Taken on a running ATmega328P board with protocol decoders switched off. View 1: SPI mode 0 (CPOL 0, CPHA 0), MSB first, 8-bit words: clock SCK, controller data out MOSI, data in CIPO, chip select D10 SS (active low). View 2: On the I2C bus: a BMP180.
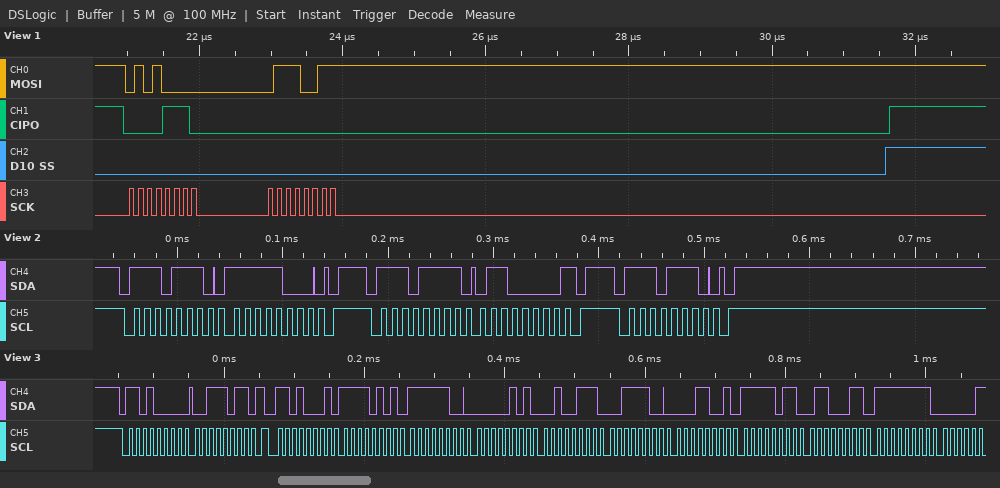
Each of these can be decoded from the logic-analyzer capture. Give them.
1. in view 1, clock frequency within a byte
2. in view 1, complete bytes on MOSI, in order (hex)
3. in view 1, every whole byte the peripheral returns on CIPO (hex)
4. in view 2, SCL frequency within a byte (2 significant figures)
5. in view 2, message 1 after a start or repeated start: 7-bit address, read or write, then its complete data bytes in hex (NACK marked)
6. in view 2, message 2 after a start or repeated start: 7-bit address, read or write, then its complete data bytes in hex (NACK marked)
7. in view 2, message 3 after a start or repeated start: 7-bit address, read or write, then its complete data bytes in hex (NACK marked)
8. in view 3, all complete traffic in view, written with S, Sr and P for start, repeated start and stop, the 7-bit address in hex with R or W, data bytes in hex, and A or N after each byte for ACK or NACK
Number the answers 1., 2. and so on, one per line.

1. 8 MHz
2. 50 73
3. 0E 00
4. 100 kHz
5. 0x77 write: F8
6. 0x77 read: 60 NACK
7. 0x77 write
8. S 68W A 3B A Sr 68R A F5 A FC A 05 A 27 A 3C A 19 A FB A 63 A FF A
